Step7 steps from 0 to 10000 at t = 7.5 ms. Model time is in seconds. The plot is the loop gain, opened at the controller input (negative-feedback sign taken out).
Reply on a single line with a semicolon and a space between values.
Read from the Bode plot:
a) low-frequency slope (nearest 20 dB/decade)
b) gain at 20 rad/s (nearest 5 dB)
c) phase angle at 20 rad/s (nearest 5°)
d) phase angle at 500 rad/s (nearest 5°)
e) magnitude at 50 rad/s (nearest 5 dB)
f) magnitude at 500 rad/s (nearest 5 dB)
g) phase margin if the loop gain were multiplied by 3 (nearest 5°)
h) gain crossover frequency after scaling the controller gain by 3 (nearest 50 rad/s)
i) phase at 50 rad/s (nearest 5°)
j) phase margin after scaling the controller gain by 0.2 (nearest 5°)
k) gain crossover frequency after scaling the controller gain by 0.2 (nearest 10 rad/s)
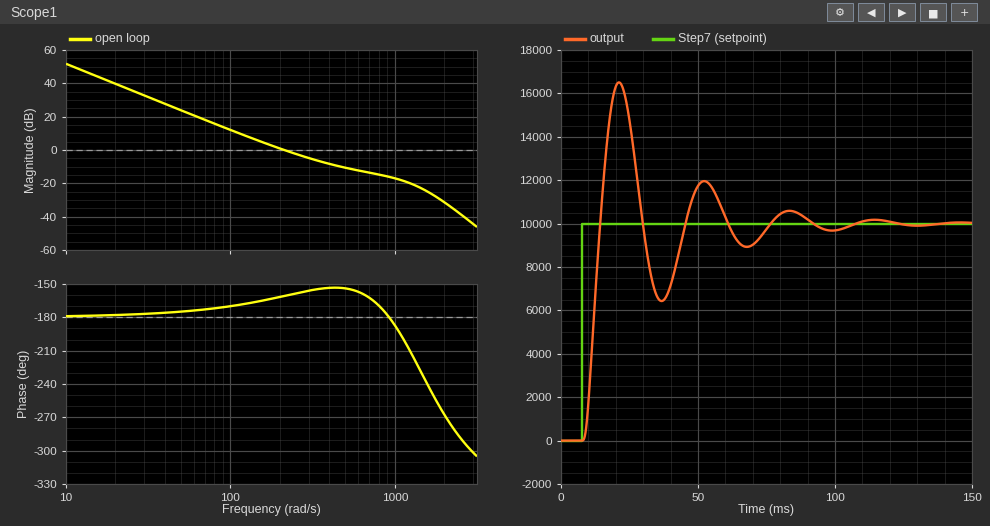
-40 dB/decade; 40 dB; -180°; -155°; 25 dB; -10 dB; 25°; 450 rad/s; -175°; 10°; 90 rad/s
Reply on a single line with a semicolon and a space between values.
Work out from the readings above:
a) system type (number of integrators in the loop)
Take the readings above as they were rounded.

2
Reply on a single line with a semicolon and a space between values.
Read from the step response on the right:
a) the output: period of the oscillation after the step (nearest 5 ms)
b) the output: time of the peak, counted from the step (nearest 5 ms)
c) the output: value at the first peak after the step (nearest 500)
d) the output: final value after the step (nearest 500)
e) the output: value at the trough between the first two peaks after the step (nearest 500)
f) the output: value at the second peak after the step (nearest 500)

30 ms; 15 ms; 16500; 10000; 6500; 12000
